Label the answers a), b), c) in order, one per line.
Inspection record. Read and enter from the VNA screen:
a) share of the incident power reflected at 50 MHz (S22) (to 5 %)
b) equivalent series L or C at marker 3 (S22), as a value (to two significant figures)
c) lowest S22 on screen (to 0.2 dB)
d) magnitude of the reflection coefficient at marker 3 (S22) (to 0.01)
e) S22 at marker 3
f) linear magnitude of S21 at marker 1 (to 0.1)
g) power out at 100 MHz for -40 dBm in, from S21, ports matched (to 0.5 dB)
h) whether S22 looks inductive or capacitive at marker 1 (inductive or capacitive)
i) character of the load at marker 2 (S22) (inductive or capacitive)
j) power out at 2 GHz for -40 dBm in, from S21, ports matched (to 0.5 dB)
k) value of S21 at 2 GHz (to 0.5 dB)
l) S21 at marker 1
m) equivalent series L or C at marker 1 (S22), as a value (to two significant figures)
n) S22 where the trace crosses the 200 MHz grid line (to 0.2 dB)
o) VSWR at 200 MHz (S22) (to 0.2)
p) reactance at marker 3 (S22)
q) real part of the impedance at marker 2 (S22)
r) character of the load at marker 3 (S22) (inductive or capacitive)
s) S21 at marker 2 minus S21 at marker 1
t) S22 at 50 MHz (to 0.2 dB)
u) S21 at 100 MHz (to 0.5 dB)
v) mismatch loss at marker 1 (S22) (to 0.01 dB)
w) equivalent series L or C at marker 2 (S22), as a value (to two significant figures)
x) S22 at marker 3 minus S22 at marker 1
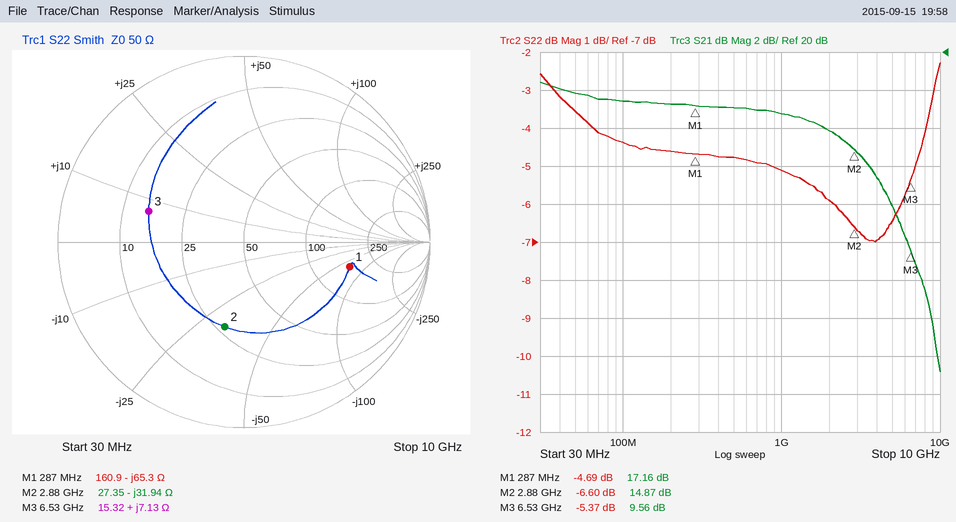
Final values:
a) 45 %
b) 170 pH
c) -7.0 dB
d) 0.54
e) -5.37 dB
f) 7.2
g) -22.5 dBm
h) capacitive
i) capacitive
j) -24.0 dBm
k) 16.0 dB
l) 17.16 dB
m) 8.5 pF
n) -4.6 dB
o) 3.8
p) +7.13 Ω
q) 27.35 Ω
r) inductive
s) -2.29 dB
t) -3.6 dB
u) 17.5 dB
v) 1.80 dB
w) 1.7 pF
x) -0.68 dB
